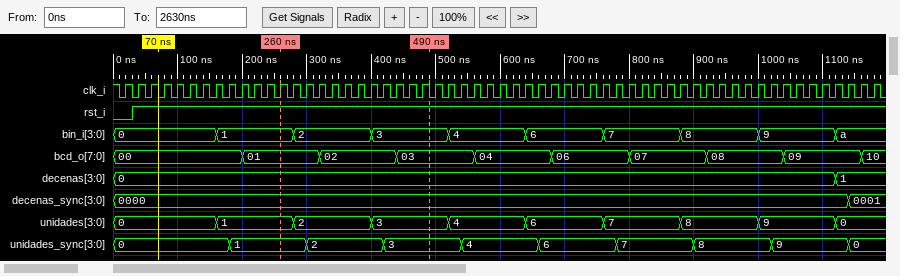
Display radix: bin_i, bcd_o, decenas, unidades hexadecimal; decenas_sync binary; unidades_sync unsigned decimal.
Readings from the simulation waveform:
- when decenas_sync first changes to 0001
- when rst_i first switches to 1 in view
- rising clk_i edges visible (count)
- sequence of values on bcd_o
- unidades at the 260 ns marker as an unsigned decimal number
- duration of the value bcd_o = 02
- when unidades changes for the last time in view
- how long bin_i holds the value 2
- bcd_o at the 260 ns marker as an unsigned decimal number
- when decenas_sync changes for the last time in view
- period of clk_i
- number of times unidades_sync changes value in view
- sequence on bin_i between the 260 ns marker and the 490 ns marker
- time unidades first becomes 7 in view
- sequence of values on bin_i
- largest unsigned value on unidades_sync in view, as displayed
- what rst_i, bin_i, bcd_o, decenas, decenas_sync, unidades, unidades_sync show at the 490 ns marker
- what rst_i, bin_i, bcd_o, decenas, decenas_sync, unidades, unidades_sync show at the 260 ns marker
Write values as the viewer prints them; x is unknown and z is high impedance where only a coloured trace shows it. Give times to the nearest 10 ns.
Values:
1140 ns
30 ns
59
00, 01, 02, 03, 04, 06, 07, 08, 09, 10
1
120 ns
1120 ns
120 ns
1
1140 ns
20 ns
9
1, 2, 3
760 ns
0, 1, 2, 3, 4, 6, 7, 8, 9, a
9
rst_i=1, bin_i=3, bcd_o=03, decenas=0, decenas_sync=0000, unidades=3, unidades_sync=3
rst_i=1, bin_i=1, bcd_o=01, decenas=0, decenas_sync=0000, unidades=1, unidades_sync=1
